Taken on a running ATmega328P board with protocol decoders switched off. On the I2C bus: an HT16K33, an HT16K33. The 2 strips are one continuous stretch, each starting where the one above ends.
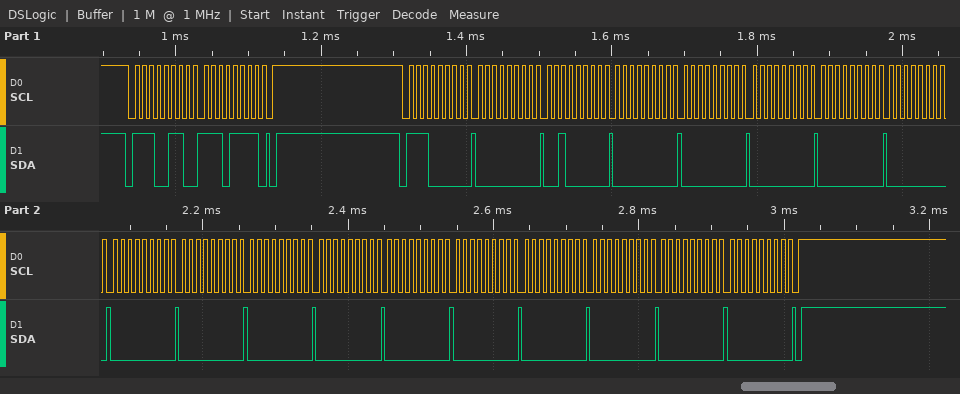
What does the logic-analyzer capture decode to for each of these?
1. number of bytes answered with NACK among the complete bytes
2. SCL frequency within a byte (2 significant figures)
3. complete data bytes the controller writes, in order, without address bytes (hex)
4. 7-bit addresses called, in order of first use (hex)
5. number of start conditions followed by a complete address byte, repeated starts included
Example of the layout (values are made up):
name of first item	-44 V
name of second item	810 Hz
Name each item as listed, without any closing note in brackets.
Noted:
number of bytes answered with NACK among the complete bytes	0
SCL frequency within a byte	100 kHz
complete data bytes the controller writes, in order, without address bytes	EF 00 20 00 00 00 00 00 00 00 00 00 00 00 00 00 00 00
7-bit addresses called, in order of first use	0x73 0x70
number of start conditions followed by a complete address byte, repeated starts included	2
